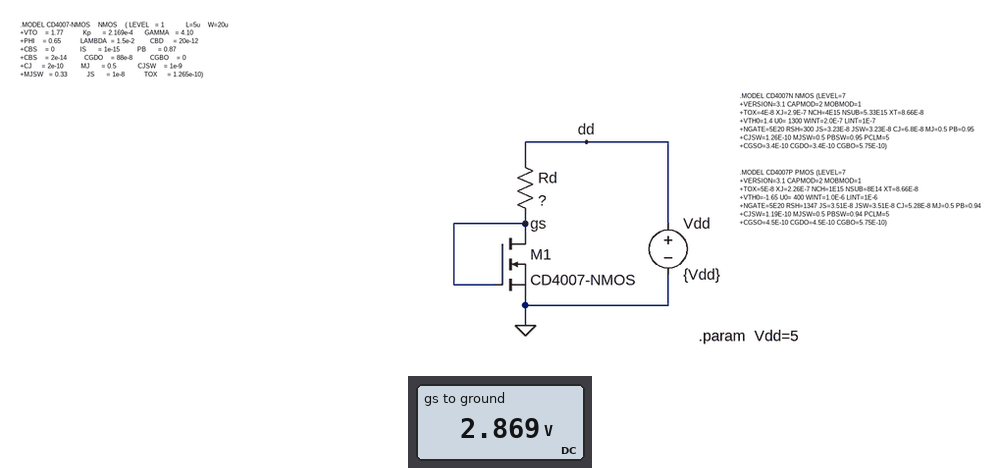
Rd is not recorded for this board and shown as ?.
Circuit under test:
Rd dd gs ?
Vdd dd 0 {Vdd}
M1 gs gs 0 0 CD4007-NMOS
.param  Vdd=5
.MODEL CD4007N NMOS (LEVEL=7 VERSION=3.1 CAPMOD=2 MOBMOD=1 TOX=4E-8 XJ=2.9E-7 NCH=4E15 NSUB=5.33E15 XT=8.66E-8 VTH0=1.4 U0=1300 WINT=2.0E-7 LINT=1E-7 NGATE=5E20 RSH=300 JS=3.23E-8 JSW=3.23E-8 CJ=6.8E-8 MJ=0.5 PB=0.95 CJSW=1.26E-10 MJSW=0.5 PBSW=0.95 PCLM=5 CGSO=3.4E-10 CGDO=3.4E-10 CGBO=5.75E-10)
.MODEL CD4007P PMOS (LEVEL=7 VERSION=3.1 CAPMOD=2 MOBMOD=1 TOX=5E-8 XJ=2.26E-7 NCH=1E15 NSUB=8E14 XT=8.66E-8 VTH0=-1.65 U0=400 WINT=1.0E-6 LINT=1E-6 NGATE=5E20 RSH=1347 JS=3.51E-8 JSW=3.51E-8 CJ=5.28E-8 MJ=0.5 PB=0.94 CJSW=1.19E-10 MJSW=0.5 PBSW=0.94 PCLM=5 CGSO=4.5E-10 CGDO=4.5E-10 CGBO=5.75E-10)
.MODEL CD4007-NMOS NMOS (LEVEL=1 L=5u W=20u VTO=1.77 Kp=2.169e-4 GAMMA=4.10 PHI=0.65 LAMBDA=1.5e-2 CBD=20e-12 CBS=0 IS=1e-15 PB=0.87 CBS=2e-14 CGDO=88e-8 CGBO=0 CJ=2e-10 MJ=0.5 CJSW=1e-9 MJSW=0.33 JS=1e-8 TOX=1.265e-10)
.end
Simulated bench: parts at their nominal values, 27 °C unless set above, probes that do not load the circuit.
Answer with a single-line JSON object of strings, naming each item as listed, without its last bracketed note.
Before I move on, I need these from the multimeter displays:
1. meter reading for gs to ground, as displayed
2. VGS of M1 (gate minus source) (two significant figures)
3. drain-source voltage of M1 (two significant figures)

{"meter reading for gs to ground, as displayed": "2.869 V", "VGS of M1 (gate minus source)": "2.9 V", "drain-source voltage of M1": "2.9 V"}
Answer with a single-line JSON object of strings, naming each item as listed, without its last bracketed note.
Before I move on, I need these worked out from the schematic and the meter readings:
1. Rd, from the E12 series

{"Rd, from the E12 series": "3.9 kΩ"}
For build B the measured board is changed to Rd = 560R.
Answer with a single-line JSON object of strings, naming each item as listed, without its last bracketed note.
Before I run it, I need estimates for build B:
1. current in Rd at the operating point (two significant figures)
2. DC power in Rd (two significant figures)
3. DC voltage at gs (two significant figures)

{"current in Rd at the operating point": "2.0 mA", "DC power in Rd": "2.3 mW", "DC voltage at gs": "3.9 V"}
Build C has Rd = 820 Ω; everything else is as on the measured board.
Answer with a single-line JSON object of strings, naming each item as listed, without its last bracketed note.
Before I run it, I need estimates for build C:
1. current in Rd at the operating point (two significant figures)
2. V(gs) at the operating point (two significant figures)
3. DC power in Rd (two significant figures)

{"current in Rd at the operating point": "1.6 mA", "V(gs) at the operating point": "3.7 V", "DC power in Rd": "2.2 mW"}
